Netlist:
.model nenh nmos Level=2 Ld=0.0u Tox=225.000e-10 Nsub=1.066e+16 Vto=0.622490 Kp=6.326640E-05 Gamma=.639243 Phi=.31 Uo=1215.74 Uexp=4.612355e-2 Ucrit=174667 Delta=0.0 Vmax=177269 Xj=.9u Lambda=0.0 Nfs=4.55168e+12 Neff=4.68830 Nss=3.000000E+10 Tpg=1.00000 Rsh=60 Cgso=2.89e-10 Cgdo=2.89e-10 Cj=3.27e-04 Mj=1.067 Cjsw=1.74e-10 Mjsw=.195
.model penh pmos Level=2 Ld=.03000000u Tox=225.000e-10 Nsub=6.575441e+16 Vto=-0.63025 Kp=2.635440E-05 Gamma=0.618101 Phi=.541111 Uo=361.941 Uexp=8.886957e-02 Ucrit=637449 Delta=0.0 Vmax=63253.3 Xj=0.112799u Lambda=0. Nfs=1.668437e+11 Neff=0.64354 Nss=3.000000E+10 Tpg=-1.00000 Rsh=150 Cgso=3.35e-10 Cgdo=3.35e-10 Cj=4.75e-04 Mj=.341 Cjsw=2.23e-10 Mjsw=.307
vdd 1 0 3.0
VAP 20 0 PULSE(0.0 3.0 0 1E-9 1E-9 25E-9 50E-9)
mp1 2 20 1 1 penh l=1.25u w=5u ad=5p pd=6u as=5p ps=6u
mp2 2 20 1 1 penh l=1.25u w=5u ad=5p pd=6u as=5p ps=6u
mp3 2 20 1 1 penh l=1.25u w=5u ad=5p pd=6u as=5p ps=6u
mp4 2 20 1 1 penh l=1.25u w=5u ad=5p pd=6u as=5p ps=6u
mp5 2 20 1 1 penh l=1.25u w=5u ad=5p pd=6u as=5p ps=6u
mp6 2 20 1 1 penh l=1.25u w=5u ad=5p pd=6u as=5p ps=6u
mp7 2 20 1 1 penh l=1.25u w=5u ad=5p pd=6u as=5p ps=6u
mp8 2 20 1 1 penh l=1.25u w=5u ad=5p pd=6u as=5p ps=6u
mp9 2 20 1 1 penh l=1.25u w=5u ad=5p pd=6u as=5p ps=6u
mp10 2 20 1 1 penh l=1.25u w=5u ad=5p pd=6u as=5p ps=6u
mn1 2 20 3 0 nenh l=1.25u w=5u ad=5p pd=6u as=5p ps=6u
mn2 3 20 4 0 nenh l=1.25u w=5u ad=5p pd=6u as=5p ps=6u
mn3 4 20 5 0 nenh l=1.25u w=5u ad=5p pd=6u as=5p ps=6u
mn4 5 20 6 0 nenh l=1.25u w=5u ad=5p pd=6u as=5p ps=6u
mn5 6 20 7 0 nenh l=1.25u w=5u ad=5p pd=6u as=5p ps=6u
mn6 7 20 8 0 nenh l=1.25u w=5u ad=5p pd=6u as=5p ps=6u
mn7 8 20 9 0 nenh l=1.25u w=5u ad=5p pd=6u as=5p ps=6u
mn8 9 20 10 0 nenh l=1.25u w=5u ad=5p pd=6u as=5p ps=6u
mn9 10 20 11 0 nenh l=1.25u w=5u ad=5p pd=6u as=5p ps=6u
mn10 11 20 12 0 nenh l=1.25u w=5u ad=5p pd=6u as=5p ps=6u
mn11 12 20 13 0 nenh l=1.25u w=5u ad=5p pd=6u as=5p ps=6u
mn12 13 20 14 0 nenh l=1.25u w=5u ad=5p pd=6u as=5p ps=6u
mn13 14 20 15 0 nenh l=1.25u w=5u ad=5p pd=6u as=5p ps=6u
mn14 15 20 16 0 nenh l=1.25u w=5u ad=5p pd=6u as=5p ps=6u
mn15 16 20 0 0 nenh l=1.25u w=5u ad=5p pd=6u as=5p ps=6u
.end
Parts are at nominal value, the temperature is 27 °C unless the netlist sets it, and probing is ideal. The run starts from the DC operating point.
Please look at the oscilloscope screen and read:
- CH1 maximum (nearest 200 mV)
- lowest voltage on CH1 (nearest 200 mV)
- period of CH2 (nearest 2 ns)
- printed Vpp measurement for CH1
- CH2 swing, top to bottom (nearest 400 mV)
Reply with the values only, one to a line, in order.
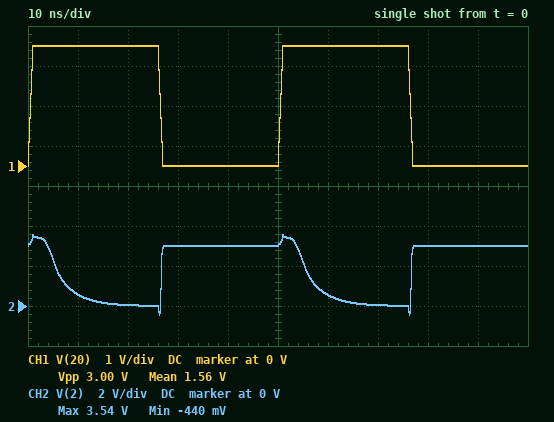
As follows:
3.0 V
0 V
50 ns
3.00 V
4.0 V
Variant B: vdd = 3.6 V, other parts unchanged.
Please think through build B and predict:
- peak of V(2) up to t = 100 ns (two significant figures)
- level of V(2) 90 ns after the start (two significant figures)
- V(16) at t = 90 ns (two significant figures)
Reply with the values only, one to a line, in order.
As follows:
3.9 V
3.6 V
-210 mV
